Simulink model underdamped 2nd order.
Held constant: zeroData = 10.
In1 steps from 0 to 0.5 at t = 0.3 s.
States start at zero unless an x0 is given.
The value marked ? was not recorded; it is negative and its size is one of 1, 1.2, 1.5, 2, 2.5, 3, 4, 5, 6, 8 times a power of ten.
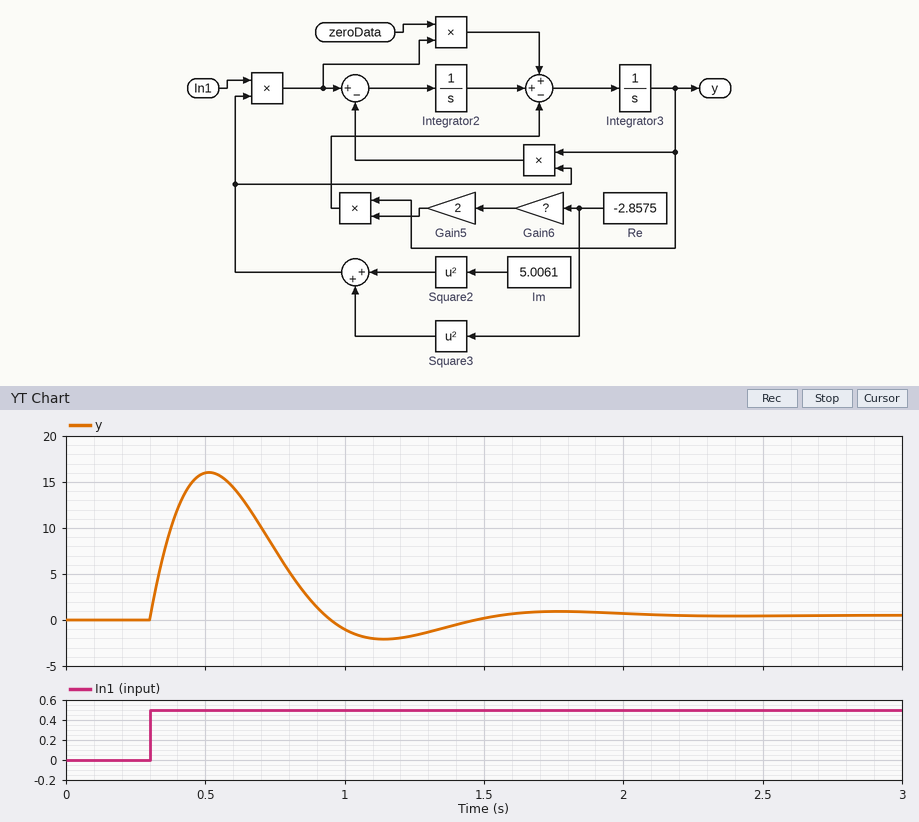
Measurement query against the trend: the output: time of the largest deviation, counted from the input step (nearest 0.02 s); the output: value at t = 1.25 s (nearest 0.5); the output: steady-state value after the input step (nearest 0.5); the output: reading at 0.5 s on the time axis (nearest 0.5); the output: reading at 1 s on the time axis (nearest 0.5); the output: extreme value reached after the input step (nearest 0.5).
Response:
0.22 s
-1.5
0.5
16.0
-1.0
16.0
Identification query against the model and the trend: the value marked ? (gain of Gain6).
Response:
-1
